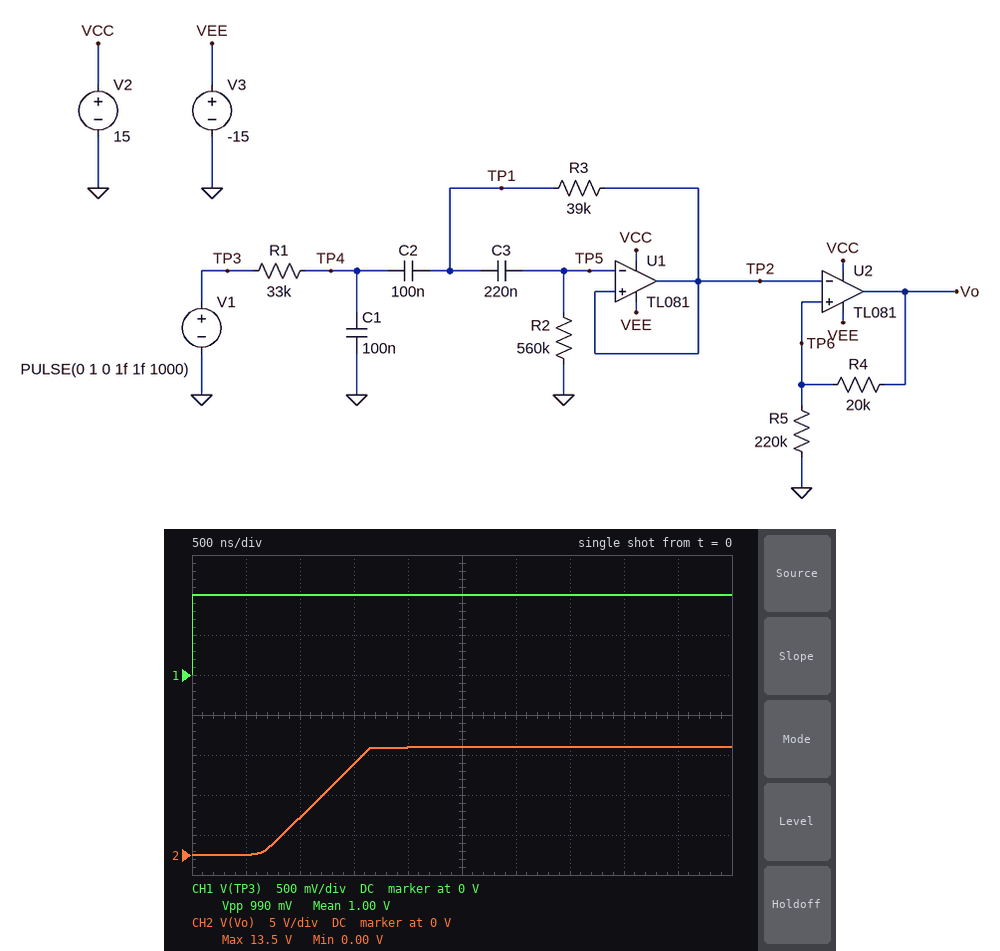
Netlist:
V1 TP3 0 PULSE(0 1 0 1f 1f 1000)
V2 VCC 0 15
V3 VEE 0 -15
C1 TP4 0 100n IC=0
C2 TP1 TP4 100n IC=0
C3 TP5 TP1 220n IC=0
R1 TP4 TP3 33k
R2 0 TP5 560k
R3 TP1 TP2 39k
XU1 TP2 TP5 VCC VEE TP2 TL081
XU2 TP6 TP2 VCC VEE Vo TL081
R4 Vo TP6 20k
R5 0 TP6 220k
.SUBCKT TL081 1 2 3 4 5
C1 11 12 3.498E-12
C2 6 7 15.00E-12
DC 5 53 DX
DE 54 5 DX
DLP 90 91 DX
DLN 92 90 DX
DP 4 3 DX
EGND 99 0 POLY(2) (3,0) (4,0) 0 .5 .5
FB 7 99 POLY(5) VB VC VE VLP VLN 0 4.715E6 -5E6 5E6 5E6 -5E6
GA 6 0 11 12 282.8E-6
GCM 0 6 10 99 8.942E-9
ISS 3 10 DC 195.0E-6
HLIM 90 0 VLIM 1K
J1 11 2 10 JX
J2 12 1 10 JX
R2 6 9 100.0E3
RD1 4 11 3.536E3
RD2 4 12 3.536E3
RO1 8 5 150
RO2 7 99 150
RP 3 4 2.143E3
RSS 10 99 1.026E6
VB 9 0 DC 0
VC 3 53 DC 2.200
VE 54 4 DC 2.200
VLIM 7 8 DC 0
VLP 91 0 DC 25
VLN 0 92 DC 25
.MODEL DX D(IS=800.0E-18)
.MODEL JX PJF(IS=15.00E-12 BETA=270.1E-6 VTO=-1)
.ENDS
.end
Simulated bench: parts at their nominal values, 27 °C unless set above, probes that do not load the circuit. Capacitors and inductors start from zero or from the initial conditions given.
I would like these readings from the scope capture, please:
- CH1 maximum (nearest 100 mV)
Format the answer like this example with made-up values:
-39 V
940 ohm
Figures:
1.0 V
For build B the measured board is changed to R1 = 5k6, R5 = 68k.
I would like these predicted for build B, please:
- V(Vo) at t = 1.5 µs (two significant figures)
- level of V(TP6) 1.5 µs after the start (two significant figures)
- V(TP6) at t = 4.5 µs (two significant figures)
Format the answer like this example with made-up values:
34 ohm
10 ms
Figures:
13 V
10 V
10 V
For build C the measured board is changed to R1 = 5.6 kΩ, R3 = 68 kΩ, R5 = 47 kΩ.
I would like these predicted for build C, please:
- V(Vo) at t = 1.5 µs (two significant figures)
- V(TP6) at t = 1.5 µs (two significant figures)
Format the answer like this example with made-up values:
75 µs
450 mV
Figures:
13 V
9.4 V
